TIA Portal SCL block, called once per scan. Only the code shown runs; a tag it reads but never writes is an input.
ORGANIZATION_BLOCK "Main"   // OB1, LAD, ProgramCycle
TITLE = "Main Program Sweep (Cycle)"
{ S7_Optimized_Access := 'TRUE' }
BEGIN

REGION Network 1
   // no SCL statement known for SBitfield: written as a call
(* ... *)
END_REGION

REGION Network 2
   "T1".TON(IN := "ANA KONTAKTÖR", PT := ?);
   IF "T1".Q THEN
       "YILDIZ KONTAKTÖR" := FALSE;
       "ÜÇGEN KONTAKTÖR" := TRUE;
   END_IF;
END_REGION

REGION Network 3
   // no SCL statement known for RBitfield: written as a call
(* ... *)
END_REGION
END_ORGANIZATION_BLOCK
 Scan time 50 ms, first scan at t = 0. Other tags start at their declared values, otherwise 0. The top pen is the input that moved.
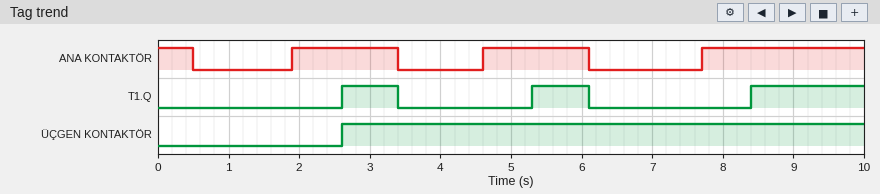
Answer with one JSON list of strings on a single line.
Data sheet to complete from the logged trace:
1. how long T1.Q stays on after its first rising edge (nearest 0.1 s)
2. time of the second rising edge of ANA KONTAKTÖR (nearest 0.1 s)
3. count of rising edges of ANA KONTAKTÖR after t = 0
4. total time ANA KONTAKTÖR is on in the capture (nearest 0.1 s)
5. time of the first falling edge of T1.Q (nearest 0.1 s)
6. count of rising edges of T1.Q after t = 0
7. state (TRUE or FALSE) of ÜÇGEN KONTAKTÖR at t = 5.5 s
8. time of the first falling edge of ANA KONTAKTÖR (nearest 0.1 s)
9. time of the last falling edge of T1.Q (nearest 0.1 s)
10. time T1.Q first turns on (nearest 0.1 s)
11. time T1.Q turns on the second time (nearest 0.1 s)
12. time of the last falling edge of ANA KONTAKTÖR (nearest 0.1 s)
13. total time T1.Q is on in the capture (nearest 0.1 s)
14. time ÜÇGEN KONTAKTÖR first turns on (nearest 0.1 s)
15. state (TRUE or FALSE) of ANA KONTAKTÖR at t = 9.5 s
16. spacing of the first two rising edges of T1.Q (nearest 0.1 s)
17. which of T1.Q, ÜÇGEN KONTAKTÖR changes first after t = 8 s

["0.8 s", "4.6 s", "3", "5.8 s", "3.4 s", "3", "TRUE", "0.5 s", "6.1 s", "2.6 s", "5.3 s", "6.1 s", "3.2 s", "2.6 s", "TRUE", "2.7 s", "T1.Q"]
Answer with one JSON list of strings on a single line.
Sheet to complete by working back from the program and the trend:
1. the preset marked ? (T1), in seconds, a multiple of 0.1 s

["0.7 s"]
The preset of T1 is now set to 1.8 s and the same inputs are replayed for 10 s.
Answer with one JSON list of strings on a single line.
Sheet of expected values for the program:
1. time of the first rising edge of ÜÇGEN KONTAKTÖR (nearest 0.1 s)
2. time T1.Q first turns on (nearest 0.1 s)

["9.5 s", "9.5 s"]
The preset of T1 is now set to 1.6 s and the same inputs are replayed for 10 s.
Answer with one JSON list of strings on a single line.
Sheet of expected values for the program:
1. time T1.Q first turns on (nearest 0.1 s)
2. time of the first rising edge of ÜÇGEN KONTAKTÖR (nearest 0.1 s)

["9.3 s", "9.3 s"]
